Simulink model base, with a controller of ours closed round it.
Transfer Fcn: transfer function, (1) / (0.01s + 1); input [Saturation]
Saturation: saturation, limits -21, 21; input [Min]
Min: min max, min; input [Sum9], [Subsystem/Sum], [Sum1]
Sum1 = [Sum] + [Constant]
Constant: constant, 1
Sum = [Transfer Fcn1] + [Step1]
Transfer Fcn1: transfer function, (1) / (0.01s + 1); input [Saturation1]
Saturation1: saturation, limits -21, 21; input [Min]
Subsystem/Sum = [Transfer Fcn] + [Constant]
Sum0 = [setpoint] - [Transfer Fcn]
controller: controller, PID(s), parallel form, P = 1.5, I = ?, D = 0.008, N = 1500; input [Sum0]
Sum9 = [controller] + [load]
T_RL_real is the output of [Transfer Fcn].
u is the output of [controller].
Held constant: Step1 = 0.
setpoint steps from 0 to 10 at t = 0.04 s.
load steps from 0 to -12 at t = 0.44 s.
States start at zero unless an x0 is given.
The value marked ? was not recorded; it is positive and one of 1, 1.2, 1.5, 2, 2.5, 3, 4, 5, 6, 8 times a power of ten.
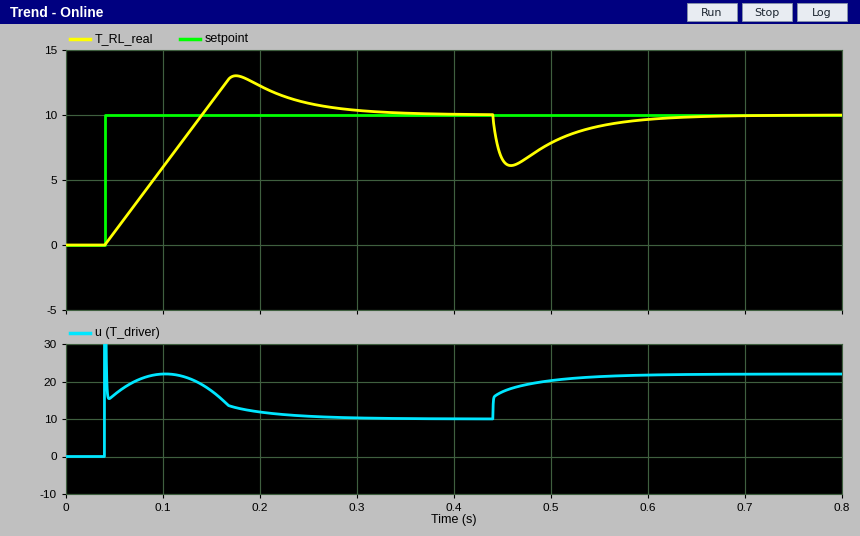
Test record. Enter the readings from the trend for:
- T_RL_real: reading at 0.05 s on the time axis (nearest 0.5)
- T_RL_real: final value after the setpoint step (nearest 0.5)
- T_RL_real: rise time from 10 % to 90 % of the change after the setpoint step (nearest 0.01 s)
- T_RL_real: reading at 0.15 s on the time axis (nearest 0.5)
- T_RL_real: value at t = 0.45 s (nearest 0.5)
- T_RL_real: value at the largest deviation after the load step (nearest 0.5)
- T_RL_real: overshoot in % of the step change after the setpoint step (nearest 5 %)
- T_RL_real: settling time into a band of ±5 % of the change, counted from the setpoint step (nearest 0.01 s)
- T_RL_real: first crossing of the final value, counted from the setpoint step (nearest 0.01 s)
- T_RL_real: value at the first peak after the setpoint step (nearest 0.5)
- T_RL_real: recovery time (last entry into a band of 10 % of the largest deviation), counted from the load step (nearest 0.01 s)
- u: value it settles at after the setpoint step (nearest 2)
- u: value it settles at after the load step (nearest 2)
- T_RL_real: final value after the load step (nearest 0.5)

1.0
10.0
0.08 s
11.0
6.5
6.0
30 %
0.24 s
0.10 s
13.0
0.15 s
10
22
10.0
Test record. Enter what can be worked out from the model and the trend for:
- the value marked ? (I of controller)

40
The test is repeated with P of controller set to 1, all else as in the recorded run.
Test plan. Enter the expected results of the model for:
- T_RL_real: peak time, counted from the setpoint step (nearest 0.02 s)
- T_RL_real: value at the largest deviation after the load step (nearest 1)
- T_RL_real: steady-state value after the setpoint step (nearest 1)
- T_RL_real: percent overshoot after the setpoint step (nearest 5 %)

0.14 s
5
10
35 %
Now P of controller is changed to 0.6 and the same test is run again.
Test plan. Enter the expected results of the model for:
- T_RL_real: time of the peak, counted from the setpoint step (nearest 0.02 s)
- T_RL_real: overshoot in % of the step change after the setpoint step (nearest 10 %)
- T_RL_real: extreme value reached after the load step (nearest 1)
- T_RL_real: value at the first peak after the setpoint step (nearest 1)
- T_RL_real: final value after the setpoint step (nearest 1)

0.14 s
40 %
5
14
10
